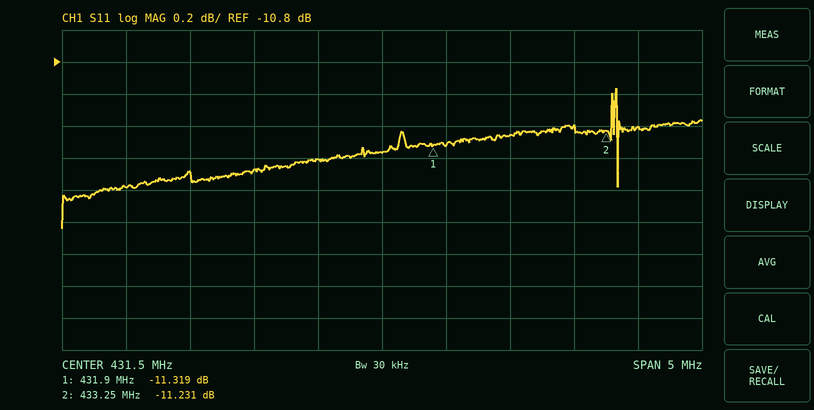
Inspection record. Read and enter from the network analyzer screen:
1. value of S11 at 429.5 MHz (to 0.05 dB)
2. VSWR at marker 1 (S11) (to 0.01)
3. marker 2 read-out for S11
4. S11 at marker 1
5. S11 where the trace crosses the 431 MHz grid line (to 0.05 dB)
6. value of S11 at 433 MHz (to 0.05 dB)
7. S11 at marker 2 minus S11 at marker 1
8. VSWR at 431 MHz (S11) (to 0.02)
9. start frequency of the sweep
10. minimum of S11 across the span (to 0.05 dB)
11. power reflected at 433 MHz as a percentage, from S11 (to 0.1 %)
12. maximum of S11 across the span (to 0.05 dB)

-11.60 dB
1.75
-11.231 dB
-11.319 dB
-11.40 dB
-11.20 dB
0.088 dB
1.74
429 MHz
-11.85 dB
7.6 %
-10.95 dB
